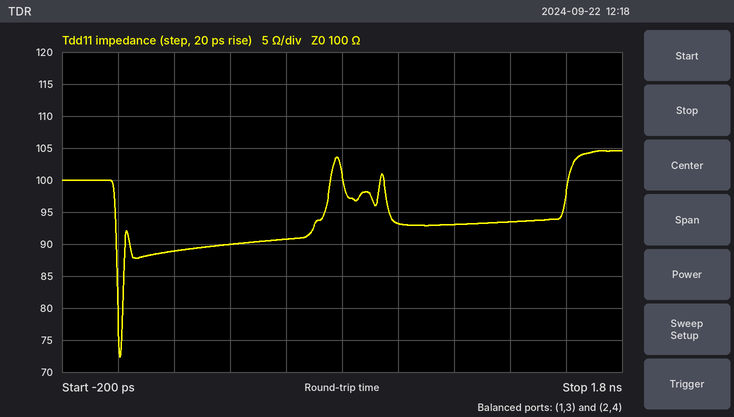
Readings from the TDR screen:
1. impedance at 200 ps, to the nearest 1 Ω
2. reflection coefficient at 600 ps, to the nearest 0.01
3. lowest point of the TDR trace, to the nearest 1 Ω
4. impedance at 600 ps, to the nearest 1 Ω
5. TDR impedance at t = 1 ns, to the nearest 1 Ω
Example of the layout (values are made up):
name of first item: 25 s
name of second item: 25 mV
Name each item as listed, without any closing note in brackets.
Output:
impedance at 200 ps, to the nearest 1 Ω: 89 Ω
reflection coefficient at 600 ps, to the nearest 0.01: -0.05
lowest point of the TDR trace, to the nearest 1 Ω: 72 Ω
impedance at 600 ps, to the nearest 1 Ω: 91 Ω
TDR impedance at t = 1 ns, to the nearest 1 Ω: 93 Ω
